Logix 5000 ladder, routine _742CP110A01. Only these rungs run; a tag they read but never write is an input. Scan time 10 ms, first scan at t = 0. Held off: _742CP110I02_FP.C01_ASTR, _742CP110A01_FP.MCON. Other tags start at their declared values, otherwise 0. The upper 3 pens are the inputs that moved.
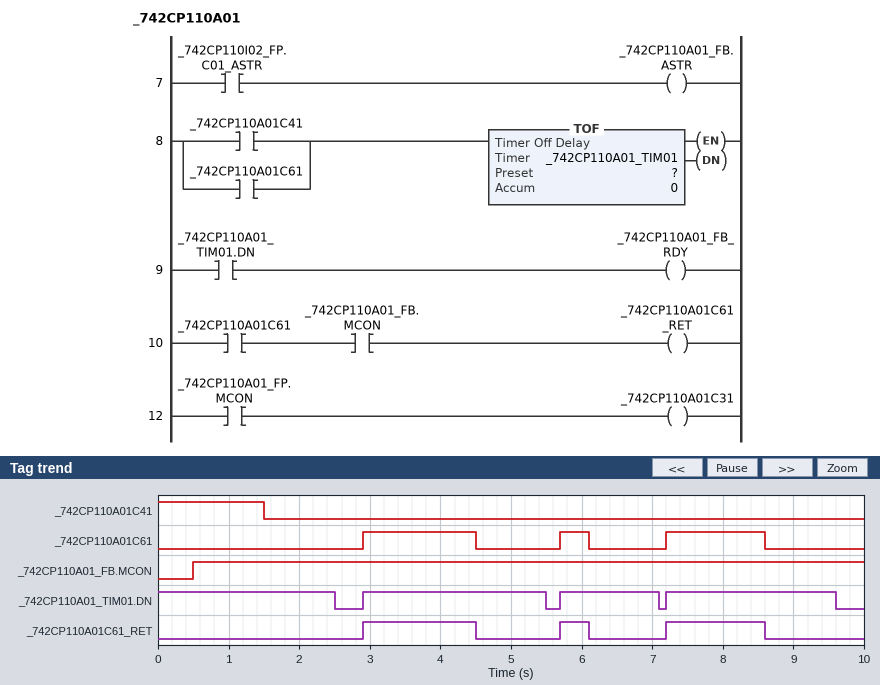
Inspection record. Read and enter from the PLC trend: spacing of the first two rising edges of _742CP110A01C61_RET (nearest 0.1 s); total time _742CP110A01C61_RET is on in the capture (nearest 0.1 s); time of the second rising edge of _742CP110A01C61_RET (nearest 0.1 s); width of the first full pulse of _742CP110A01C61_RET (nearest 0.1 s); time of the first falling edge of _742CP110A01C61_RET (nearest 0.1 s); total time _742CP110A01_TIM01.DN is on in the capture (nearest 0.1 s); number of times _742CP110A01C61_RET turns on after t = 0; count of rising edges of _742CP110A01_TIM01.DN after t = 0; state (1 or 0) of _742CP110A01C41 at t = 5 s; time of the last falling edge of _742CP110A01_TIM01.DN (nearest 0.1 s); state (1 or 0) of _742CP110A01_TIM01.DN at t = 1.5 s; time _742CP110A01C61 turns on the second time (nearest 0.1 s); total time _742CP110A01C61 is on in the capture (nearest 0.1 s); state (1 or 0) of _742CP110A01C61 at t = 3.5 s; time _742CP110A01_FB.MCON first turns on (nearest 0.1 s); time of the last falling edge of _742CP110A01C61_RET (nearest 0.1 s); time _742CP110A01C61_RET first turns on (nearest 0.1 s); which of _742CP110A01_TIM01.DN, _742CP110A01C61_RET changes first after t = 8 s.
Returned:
2.8 s
3.4 s
5.7 s
1.6 s
4.5 s
8.9 s
3
3
0
9.6 s
1
5.7 s
3.4 s
1
0.5 s
8.6 s
2.9 s
_742CP110A01C61_RET
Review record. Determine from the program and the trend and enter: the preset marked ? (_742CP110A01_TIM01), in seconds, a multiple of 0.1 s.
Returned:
1.0 s
